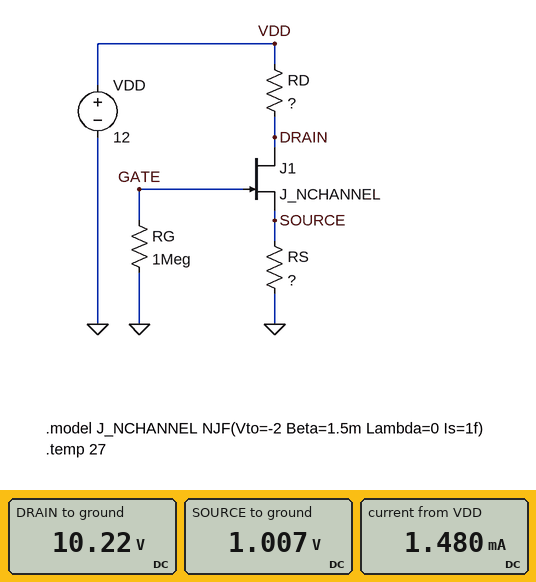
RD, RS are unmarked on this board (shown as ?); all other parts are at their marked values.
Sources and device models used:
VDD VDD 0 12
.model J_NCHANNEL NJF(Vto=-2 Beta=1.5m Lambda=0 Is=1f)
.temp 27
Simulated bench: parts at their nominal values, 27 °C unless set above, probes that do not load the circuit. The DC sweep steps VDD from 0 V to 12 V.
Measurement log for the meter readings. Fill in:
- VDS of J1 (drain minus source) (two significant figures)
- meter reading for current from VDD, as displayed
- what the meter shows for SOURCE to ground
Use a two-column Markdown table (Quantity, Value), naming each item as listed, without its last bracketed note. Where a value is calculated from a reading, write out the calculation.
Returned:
| Quantity | Value |
|---|---|
| VDS of J1 (drain minus source) | 10.22 V - 1.007 V = 9.2 V |
| meter reading for current from VDD, as displayed | 1.480 mA |
| what the meter shows for SOURCE to ground | 1.007 V |
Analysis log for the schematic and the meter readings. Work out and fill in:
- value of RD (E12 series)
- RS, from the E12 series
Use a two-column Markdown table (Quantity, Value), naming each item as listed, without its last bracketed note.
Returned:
| Quantity | Value |
|---|---|
| value of RD | 1.2 kΩ |
| RS, from the E12 series | 680 Ω |
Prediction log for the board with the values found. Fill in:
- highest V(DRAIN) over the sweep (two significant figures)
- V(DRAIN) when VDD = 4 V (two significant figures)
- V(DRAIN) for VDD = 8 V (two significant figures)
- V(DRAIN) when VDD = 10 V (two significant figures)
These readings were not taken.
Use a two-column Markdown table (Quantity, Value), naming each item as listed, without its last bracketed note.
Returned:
| Quantity | Value |
|---|---|
| highest V(DRAIN) over the sweep | 10 V |
| V(DRAIN) when VDD = 4 V | 2.2 V |
| V(DRAIN) for VDD = 8 V | 6.2 V |
| V(DRAIN) when VDD = 10 V | 8.2 V |
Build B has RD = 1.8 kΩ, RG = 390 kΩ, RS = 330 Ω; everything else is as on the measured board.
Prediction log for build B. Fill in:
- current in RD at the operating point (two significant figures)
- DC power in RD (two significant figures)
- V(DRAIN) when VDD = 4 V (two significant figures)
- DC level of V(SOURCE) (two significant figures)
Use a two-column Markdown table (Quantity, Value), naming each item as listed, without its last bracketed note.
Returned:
| Quantity | Value |
|---|---|
| current in RD at the operating point | 2.3 mA |
| DC power in RD | 9.6 mW |
| V(DRAIN) when VDD = 4 V | 1.0 V |
| DC level of V(SOURCE) | 760 mV |
